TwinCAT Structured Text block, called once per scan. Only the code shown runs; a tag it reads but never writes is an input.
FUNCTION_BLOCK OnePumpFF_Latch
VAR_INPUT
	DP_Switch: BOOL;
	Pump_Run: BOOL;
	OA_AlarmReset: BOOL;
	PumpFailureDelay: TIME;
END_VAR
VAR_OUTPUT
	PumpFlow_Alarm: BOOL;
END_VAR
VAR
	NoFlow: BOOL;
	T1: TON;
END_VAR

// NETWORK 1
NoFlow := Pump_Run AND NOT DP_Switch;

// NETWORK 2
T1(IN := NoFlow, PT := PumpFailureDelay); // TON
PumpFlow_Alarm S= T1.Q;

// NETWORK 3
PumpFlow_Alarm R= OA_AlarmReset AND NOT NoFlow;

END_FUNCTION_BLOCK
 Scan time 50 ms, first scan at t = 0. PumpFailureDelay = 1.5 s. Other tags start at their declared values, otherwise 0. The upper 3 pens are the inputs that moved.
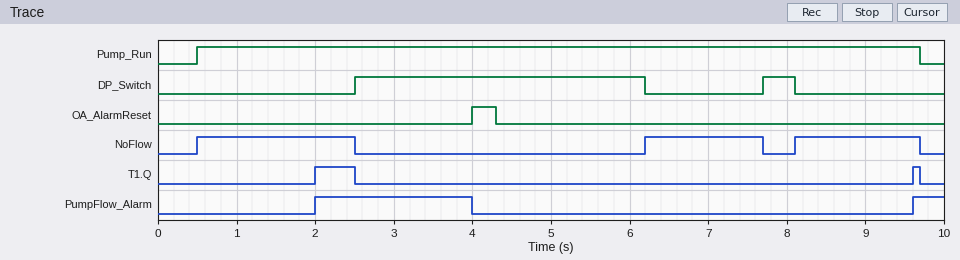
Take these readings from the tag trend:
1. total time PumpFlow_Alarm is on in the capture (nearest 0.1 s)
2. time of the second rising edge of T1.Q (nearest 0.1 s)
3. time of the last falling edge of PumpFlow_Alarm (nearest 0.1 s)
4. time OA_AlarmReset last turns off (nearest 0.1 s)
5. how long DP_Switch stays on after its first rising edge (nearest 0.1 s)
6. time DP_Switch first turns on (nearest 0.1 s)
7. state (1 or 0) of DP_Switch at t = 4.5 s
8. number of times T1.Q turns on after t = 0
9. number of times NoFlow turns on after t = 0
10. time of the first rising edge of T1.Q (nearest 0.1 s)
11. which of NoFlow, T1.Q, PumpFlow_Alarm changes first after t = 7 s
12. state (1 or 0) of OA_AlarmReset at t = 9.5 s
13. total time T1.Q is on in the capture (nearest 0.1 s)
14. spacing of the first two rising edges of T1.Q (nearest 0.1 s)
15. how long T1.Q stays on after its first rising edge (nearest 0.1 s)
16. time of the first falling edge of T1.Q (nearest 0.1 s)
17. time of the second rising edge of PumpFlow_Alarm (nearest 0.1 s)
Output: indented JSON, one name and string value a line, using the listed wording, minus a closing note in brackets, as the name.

{
  "total time PumpFlow_Alarm is on in the capture": "2.4 s",
  "time of the second rising edge of T1.Q": "9.6 s",
  "time of the last falling edge of PumpFlow_Alarm": "4.0 s",
  "time OA_AlarmReset last turns off": "4.3 s",
  "how long DP_Switch stays on after its first rising edge": "3.7 s",
  "time DP_Switch first turns on": "2.5 s",
  "state (1 or 0) of DP_Switch at t = 4.5 s": "1",
  "number of times T1.Q turns on after t = 0": "2",
  "number of times NoFlow turns on after t = 0": "3",
  "time of the first rising edge of T1.Q": "2.0 s",
  "which of NoFlow, T1.Q, PumpFlow_Alarm changes first after t = 7 s": "NoFlow",
  "state (1 or 0) of OA_AlarmReset at t = 9.5 s": "0",
  "total time T1.Q is on in the capture": "0.6 s",
  "spacing of the first two rising edges of T1.Q": "7.6 s",
  "how long T1.Q stays on after its first rising edge": "0.5 s",
  "time of the first falling edge of T1.Q": "2.5 s",
  "time of the second rising edge of PumpFlow_Alarm": "9.6 s"
}
